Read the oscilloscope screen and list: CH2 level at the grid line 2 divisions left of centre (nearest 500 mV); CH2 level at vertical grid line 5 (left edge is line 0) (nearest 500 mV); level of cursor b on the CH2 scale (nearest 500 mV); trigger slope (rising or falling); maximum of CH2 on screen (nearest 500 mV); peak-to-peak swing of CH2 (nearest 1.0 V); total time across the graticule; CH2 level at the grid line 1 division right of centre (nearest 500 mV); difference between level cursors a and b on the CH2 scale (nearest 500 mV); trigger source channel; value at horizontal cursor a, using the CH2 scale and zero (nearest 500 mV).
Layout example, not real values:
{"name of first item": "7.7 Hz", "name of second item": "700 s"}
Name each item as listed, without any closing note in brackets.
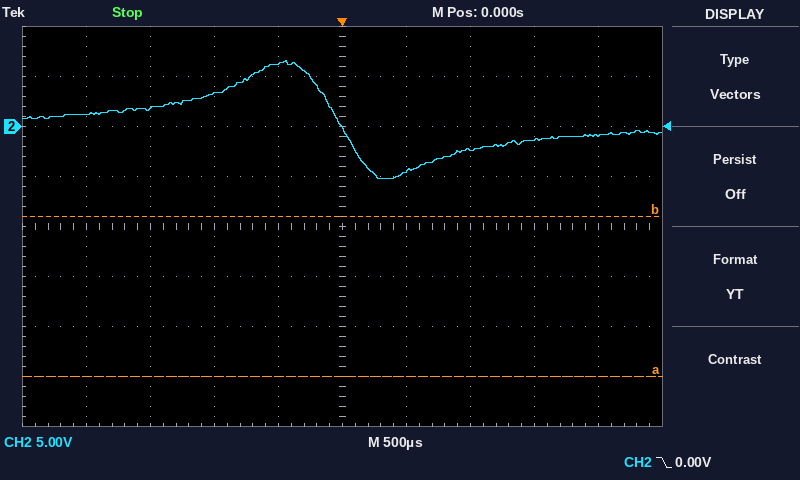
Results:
{"CH2 level at the grid line 2 divisions left of centre": "3.5 V", "CH2 level at vertical grid line 5 (left edge is line 0)": "0.0 V", "level of cursor b on the CH2 scale": "-9.0 V", "trigger slope": "falling", "maximum of CH2 on screen": "6.5 V", "peak-to-peak swing of CH2": "12.0 V", "total time across the graticule": "5 ms", "CH2 level at the grid line 1 division right of centre": "-4.5 V", "difference between level cursors a and b on the CH2 scale": "16.0 V", "trigger source channel": "CH2", "value at horizontal cursor a, using the CH2 scale and zero": "-25.0 V"}
